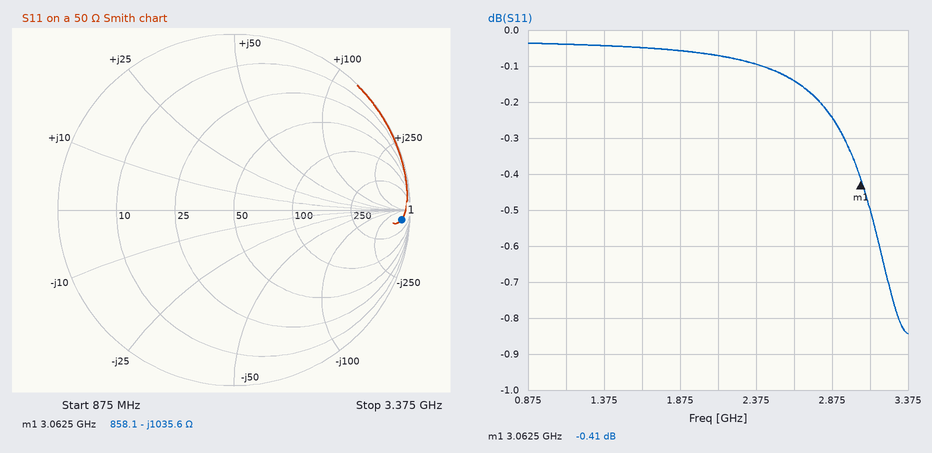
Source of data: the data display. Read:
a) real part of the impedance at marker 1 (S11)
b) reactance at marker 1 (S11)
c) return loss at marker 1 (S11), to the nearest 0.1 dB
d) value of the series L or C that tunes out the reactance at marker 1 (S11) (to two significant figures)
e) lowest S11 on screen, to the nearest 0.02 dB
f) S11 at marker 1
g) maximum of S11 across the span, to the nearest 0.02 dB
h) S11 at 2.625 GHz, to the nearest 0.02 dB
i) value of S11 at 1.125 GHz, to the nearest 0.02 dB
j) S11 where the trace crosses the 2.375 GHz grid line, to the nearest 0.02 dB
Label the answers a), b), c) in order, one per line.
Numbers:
a) 858.1 Ω
b) -1035.6 Ω
c) 0.4 dB
d) 54 nH
e) -0.84 dB
f) -0.41 dB
g) -0.04 dB
h) -0.14 dB
i) -0.04 dB
j) -0.10 dB
